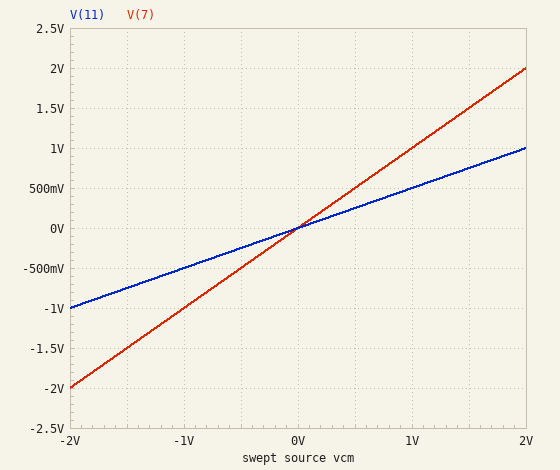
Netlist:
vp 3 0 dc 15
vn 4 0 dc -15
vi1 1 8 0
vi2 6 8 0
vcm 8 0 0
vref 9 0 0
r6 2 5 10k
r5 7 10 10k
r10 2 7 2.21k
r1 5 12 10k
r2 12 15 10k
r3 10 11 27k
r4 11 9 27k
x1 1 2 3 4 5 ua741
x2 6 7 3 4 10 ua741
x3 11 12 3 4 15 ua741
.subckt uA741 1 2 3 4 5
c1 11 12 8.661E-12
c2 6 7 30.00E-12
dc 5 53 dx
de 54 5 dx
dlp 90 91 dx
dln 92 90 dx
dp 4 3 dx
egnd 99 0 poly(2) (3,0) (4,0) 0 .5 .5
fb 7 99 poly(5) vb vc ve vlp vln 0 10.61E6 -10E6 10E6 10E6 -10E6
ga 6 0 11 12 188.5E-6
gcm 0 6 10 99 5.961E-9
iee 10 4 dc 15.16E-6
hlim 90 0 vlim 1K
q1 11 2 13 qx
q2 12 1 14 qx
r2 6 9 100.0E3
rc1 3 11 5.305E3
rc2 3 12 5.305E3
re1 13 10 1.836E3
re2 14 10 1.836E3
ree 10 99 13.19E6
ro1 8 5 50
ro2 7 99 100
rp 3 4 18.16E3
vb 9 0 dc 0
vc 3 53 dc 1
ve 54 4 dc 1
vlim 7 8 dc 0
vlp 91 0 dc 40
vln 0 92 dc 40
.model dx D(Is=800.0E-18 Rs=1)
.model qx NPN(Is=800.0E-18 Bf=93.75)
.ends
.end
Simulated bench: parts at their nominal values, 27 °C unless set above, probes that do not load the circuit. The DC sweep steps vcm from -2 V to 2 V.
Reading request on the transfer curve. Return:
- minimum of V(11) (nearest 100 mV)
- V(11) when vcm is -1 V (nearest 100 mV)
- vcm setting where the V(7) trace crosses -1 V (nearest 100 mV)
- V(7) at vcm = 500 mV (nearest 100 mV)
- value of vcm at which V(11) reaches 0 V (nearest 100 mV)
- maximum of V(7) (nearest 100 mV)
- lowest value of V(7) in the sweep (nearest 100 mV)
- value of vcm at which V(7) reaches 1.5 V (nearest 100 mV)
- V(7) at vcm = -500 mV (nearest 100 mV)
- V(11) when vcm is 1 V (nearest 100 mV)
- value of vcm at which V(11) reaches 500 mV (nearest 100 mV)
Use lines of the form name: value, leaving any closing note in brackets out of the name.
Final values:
minimum of V(11): -1.0 V
V(11) when vcm is -1 V: -500 mV
vcm setting where the V(7) trace crosses -1 V: -1.0 V
V(7) at vcm = 500 mV: 500 mV
value of vcm at which V(11) reaches 0 V: 0 V
maximum of V(7): 2.0 V
lowest value of V(7) in the sweep: -2.0 V
value of vcm at which V(7) reaches 1.5 V: 1.5 V
V(7) at vcm = -500 mV: -500 mV
V(11) when vcm is 1 V: 500 mV
value of vcm at which V(11) reaches 500 mV: 1.0 V
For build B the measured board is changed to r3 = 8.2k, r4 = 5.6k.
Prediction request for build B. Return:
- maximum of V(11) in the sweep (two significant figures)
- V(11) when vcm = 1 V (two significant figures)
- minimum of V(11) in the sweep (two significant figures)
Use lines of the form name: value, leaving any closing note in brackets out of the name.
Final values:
maximum of V(11) in the sweep: 810 mV
V(11) when vcm = 1 V: 410 mV
minimum of V(11) in the sweep: -810 mV
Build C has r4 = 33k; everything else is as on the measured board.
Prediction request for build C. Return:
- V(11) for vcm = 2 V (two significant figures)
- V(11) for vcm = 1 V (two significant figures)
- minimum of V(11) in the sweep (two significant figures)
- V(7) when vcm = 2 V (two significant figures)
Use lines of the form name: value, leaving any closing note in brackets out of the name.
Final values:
V(11) for vcm = 2 V: 1.1 V
V(11) for vcm = 1 V: 550 mV
minimum of V(11) in the sweep: -1.1 V
V(7) when vcm = 2 V: 2.0 V
